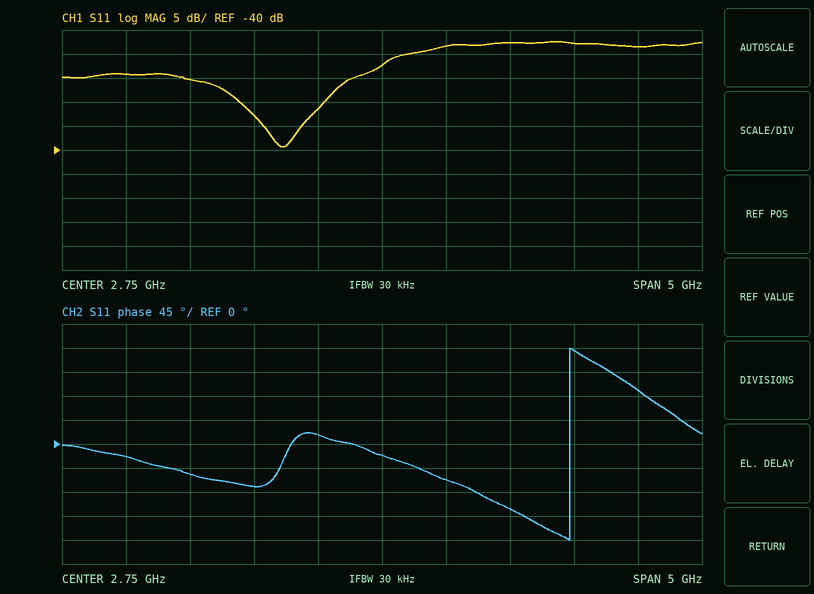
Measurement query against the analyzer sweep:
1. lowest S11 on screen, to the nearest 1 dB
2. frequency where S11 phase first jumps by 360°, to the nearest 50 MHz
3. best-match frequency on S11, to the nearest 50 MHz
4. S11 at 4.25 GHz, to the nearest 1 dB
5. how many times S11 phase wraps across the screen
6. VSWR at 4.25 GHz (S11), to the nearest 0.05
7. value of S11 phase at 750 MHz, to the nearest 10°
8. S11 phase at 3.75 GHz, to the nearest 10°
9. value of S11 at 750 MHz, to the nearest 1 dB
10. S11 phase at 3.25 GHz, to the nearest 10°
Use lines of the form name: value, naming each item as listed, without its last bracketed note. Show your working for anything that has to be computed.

lowest S11 on screen, to the nearest 1 dB: -39 dB
frequency where S11 phase first jumps by 360°, to the nearest 50 MHz: 4.20 GHz
best-match frequency on S11, to the nearest 50 MHz: 1.95 GHz
S11 at 4.25 GHz, to the nearest 1 dB: -18 dB
how many times S11 phase wraps across the screen: 1
VSWR at 4.25 GHz (S11), to the nearest 0.05: |Γ| = 10^(-18/20) = 0.1259; VSWR = (1 + 0.1259)/(1 − 0.1259) ≈ 1.29, so 1.30 to the nearest 0.05
value of S11 phase at 750 MHz, to the nearest 10°: -20°
S11 phase at 3.75 GHz, to the nearest 10°: -120°
value of S11 at 750 MHz, to the nearest 1 dB: -24 dB
S11 phase at 3.25 GHz, to the nearest 10°: -70°
